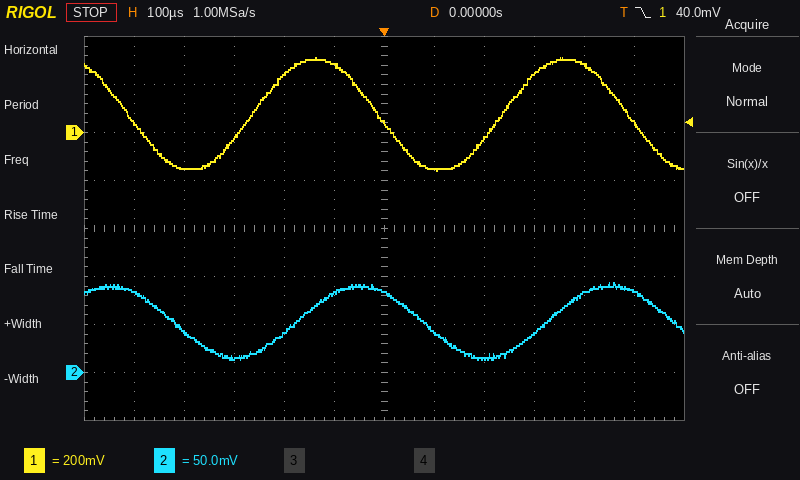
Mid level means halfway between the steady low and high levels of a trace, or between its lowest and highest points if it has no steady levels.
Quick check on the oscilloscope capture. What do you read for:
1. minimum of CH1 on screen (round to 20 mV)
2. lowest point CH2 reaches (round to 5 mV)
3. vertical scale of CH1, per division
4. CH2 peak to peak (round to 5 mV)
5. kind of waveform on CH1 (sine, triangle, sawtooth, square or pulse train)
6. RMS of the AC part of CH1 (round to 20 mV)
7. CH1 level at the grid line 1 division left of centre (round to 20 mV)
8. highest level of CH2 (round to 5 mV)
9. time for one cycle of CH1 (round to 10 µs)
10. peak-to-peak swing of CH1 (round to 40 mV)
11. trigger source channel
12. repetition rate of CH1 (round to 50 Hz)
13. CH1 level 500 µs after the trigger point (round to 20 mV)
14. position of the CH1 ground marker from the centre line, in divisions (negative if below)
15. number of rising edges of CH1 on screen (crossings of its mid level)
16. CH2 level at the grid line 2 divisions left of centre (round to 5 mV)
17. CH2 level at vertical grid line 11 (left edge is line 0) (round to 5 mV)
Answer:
-160 mV
15 mV
200 mV
80 mV
sine
160 mV
280 mV
95 mV
500 µs
480 mV
CH1
2.00 kHz
40 mV
+2.0 div
2
40 mV
85 mV
